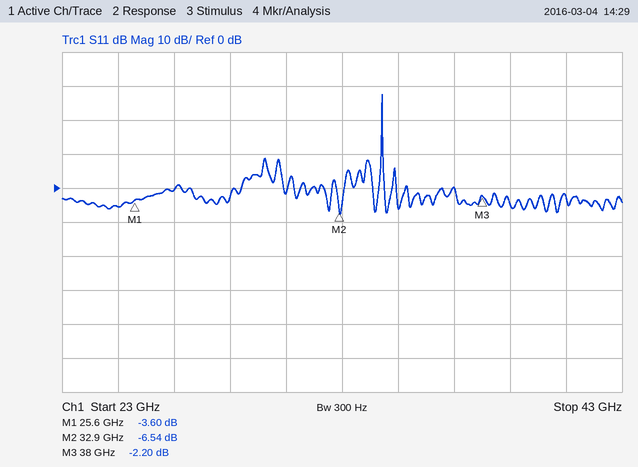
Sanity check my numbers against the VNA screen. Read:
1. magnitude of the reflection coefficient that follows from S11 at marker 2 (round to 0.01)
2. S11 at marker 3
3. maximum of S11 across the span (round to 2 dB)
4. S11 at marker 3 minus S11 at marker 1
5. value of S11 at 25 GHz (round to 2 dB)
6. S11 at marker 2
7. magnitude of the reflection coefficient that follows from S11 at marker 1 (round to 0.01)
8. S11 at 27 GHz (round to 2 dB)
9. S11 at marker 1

0.47
-2.20 dB
28 dB
1.40 dB
-6 dB
-6.54 dB
0.66
0 dB
-3.60 dB
